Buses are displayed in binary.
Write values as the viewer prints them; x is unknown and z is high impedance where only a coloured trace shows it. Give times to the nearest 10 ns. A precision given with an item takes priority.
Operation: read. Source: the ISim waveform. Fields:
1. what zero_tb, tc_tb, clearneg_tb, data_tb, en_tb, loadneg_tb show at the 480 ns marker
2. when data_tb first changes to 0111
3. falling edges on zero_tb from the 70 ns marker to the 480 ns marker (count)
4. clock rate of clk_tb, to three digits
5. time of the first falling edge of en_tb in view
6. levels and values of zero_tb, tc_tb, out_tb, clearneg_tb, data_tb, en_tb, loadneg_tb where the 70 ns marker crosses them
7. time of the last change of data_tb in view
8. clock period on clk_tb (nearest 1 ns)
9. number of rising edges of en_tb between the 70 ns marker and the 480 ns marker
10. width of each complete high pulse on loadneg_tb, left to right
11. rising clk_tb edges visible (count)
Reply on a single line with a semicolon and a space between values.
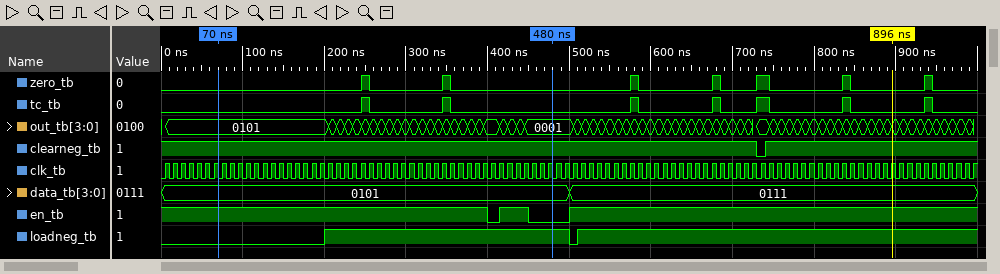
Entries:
zero_tb=0, tc_tb=0, clearneg_tb=1, data_tb=0101, en_tb=0, loadneg_tb=1; 500 ns; 2; 100 MHz; 400 ns; zero_tb=0, tc_tb=0, out_tb=0101, clearneg_tb=1, data_tb=0101, en_tb=1, loadneg_tb=0; 500 ns; 10 ns; 1; 300 ns; 100
